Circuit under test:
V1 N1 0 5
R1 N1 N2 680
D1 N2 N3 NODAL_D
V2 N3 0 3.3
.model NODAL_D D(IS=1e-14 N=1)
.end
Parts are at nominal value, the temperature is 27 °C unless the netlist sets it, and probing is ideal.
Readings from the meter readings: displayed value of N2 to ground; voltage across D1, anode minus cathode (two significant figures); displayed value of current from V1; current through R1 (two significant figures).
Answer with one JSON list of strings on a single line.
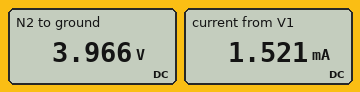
["3.966 V", "670 mV", "1.521 mA", "1.5 mA"]
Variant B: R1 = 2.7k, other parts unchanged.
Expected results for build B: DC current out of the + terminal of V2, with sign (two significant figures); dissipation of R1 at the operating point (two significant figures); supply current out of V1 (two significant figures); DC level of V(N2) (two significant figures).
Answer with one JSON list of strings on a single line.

["-400 µA", "420 µW", "400 µA", "3.9 V"]
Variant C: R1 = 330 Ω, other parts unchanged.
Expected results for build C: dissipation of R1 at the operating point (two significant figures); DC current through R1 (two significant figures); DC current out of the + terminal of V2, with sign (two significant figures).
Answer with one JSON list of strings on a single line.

["3.1 mW", "3.1 mA", "-3.1 mA"]
